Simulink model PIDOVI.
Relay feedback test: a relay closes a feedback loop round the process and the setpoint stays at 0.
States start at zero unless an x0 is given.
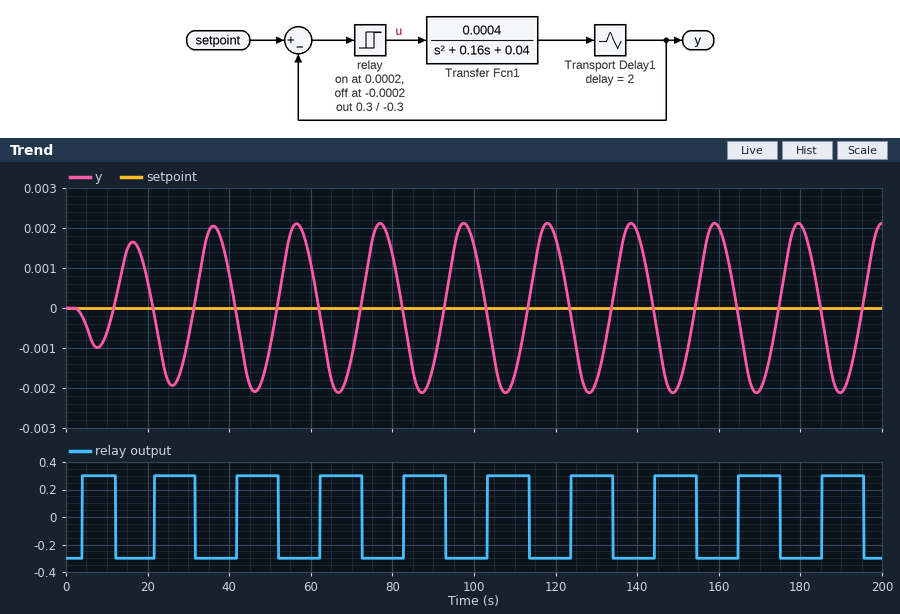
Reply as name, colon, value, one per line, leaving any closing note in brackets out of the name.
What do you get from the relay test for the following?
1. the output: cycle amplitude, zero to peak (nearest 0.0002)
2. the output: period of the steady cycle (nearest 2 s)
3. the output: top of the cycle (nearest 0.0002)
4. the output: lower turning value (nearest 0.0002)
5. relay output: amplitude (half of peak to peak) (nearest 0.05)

the output: cycle amplitude, zero to peak: 0.0022
the output: period of the steady cycle: 20 s
the output: top of the cycle: 0.0022
the output: lower turning value: -0.0022
relay output: amplitude (half of peak to peak): 0.30
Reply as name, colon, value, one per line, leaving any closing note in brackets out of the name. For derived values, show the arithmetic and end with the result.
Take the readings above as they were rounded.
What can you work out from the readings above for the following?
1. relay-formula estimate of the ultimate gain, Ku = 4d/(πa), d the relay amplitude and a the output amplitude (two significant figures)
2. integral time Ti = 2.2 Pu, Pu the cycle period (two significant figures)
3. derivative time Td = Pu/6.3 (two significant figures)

relay-formula estimate of the ultimate gain, Ku = 4d/(πa), d the relay amplitude and a the output amplitude: 4 × 0.3 / (π × 0.0022) = 170
integral time Ti = 2.2 Pu, Pu the cycle period: 2.2 × 20 = 44 s
derivative time Td = Pu/6.3: 20 / 6.3 = 3.2 s
